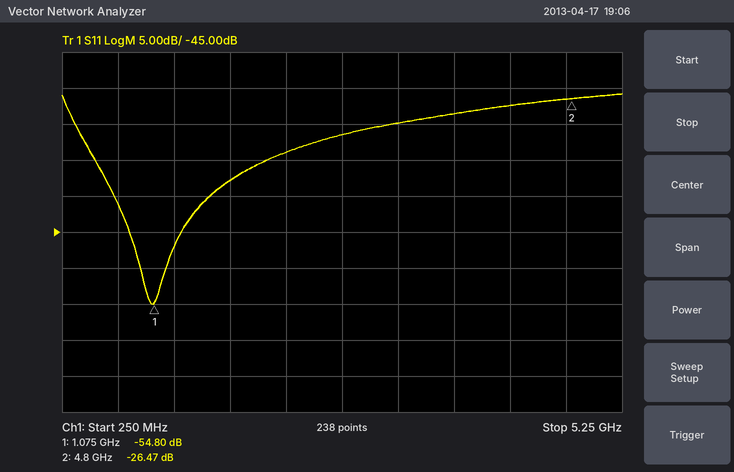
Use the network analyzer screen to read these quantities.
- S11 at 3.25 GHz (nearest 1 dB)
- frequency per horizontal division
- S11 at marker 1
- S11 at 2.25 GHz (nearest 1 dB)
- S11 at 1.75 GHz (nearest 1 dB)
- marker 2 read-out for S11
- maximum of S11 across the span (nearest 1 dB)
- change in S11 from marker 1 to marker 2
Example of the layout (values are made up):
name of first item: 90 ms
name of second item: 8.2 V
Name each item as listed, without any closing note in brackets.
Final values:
S11 at 3.25 GHz: -30 dB
frequency per horizontal division: 500 MHz
S11 at marker 1: -54.80 dB
S11 at 2.25 GHz: -34 dB
S11 at 1.75 GHz: -38 dB
marker 2 read-out for S11: -26.47 dB
maximum of S11 across the span: -26 dB
change in S11 from marker 1 to marker 2: 28.33 dB
